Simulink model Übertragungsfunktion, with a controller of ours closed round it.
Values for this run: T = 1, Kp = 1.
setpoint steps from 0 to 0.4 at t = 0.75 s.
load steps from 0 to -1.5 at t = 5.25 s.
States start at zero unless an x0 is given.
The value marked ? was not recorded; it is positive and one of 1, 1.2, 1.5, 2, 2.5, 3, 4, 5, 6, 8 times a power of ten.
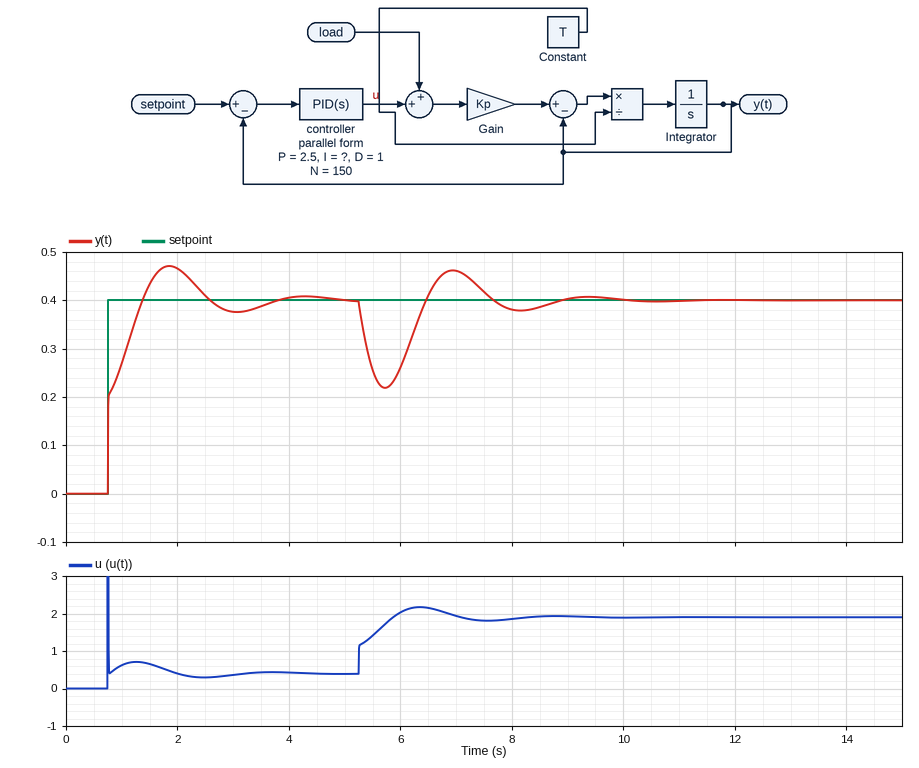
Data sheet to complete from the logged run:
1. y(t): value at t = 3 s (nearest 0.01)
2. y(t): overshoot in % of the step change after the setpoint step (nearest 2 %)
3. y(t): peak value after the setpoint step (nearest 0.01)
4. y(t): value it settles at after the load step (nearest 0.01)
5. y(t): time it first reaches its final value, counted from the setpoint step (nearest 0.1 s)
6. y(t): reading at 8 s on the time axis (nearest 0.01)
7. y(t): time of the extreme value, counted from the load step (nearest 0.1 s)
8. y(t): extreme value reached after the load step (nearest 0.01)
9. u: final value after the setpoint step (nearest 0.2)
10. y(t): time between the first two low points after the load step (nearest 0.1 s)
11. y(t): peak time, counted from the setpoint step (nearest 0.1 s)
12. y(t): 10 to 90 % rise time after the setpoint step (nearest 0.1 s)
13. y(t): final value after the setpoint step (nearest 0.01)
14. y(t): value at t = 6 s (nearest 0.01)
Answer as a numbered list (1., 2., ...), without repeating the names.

1. 0.38
2. 18 %
3. 0.47
4. 0.40
5. 0.6 s
6. 0.38
7. 0.5 s
8. 0.22
9. 0.4
10. 2.4 s
11. 1.1 s
12. 0.5 s
13. 0.40
14. 0.26
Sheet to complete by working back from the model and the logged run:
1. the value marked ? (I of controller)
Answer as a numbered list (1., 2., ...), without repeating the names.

1. 15
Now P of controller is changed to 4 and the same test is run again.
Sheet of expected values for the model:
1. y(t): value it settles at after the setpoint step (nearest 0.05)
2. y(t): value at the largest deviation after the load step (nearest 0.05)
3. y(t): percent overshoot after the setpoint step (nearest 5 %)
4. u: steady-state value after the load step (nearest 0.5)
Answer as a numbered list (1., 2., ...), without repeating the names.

1. 0.40
2. 0.25
3. 10 %
4. 2.0
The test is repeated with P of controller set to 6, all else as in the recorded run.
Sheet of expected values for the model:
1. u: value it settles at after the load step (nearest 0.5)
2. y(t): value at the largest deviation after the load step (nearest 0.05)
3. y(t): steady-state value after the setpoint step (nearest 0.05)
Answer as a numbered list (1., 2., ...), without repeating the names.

1. 2.0
2. 0.25
3. 0.40
